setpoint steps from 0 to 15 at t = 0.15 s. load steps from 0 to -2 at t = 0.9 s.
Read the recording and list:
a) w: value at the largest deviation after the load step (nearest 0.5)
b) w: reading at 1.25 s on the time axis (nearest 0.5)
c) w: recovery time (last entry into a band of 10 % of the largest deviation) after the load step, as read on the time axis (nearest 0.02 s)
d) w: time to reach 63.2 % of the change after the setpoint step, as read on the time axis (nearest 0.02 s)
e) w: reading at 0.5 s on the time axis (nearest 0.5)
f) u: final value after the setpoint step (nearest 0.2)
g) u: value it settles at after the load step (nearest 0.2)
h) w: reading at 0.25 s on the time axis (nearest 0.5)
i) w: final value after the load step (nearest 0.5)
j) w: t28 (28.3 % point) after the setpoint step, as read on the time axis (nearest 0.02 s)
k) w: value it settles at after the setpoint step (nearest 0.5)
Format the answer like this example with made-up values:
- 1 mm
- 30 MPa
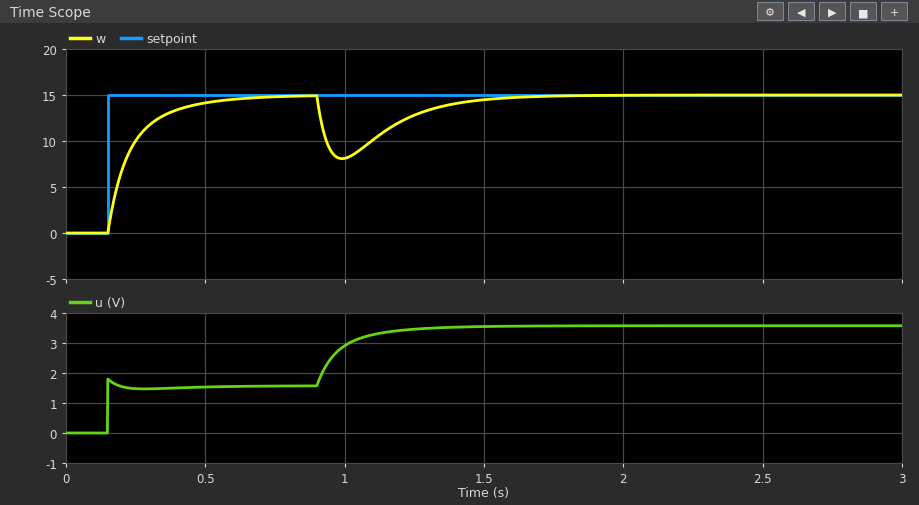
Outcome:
- 8.0
- 13.0
- 1.46 s
- 0.24 s
- 14.0
- 1.6
- 3.6
- 10.0
- 15.0
- 0.18 s
- 15.0
